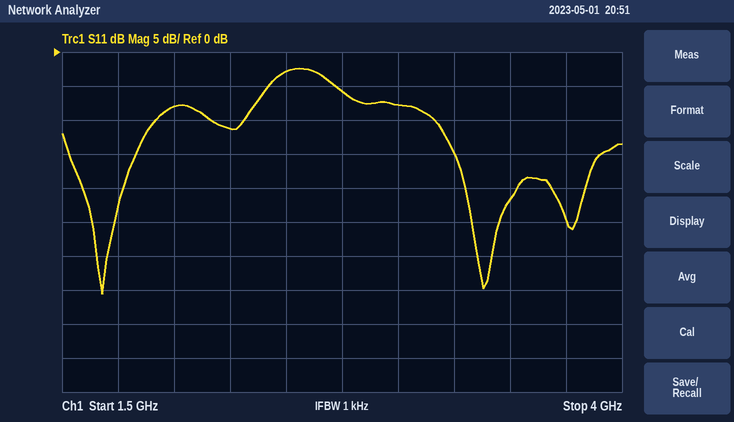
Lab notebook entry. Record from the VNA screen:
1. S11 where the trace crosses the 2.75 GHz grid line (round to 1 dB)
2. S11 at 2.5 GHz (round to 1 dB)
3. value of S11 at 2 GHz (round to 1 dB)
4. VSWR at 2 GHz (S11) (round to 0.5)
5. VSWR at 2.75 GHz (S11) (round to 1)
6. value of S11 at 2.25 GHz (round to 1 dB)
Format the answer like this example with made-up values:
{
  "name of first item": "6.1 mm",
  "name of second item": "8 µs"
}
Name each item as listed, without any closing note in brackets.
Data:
{
  "S11 where the trace crosses the 2.75 GHz grid line": "-6 dB",
  "S11 at 2.5 GHz": "-3 dB",
  "value of S11 at 2 GHz": "-8 dB",
  "VSWR at 2 GHz (S11)": "2.5",
  "VSWR at 2.75 GHz (S11)": "3",
  "value of S11 at 2.25 GHz": "-11 dB"
}
